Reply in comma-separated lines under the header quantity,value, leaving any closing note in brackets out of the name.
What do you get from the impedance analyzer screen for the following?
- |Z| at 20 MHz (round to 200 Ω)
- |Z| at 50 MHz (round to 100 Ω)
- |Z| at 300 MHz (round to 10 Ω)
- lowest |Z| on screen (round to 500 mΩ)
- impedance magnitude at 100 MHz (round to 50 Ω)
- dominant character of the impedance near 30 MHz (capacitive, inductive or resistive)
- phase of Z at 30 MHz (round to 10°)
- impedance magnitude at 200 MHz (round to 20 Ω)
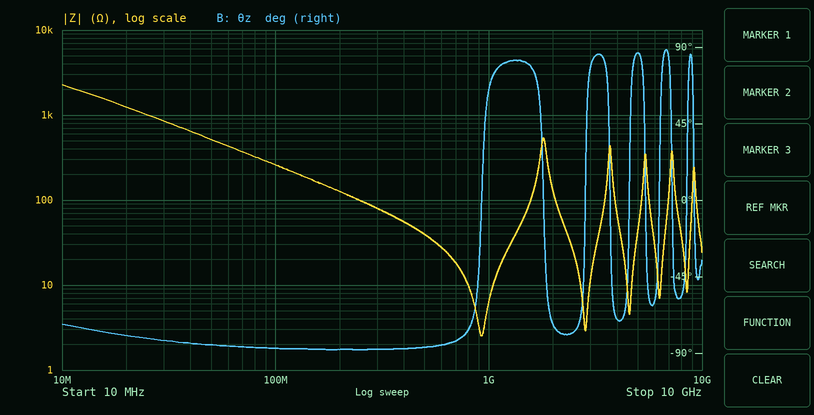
quantity,value
|Z| at 20 MHz,1.2 kΩ
|Z| at 50 MHz,500 Ω
|Z| at 300 MHz,80 Ω
lowest |Z| on screen,2.5 Ω
impedance magnitude at 100 MHz,250 Ω
dominant character of the impedance near 30 MHz,capacitive
phase of Z at 30 MHz,-80°
impedance magnitude at 200 MHz,120 Ω
